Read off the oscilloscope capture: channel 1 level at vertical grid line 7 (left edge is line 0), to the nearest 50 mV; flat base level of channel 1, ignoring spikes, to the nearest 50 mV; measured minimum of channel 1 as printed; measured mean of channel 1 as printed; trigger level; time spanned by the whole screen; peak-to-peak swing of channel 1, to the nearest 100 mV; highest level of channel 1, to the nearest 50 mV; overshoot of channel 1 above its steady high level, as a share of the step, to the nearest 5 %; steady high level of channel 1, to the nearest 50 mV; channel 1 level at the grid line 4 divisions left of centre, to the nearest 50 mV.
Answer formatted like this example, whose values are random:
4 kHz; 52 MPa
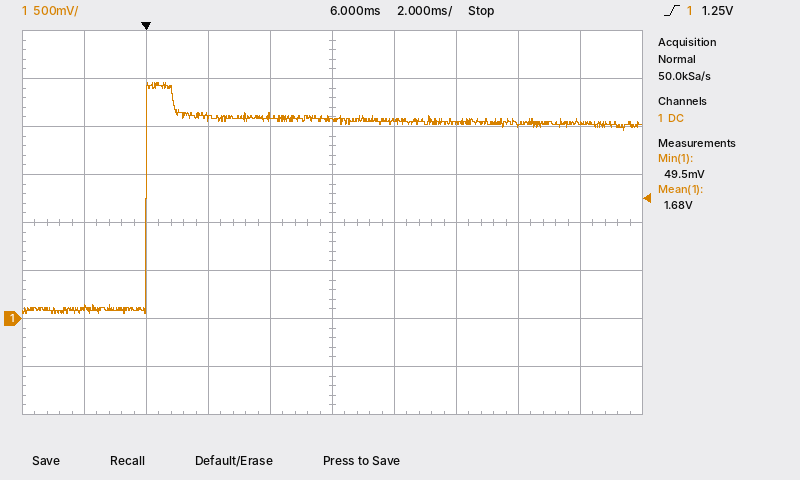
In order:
2.05 V; 100 mV; 49.5 mV; 1.68 V; 1.25 V; 20 ms; 2.40 V; 2.45 V; 20 %; 2.05 V; 100 mV
